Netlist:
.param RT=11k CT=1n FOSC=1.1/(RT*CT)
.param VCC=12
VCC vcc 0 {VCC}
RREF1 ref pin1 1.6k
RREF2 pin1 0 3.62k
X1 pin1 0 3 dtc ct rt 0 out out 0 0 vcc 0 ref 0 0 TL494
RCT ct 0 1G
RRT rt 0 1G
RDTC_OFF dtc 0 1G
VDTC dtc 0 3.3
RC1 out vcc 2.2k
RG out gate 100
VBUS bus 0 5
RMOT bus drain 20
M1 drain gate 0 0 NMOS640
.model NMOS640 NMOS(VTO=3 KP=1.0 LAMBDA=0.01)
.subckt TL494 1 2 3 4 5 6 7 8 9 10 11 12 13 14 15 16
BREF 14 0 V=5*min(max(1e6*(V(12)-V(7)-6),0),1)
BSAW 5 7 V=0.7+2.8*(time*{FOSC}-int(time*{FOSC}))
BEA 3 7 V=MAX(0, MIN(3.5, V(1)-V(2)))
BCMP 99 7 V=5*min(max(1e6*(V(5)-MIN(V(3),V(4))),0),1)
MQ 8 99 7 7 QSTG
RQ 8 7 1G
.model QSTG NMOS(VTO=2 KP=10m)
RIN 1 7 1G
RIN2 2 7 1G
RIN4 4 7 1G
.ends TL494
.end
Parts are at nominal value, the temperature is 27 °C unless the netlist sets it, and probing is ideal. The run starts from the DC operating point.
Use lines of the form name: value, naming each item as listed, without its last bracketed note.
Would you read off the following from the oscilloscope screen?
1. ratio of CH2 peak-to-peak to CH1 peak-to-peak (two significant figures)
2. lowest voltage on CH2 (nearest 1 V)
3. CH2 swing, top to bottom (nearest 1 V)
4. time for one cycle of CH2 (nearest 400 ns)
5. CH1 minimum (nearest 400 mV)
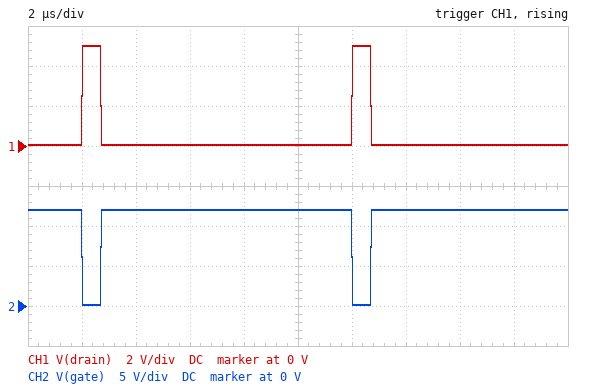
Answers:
ratio of CH2 peak-to-peak to CH1 peak-to-peak: 2.4
lowest voltage on CH2: 0 V
CH2 swing, top to bottom: 12 V
time for one cycle of CH2: 10.0 µs
CH1 minimum: 0 V
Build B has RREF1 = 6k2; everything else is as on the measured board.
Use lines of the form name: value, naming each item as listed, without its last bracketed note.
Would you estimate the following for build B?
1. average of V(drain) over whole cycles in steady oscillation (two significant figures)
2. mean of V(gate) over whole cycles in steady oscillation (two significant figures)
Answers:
average of V(drain) over whole cycles in steady oscillation: 3.0 V
mean of V(gate) over whole cycles in steady oscillation: 5.0 V
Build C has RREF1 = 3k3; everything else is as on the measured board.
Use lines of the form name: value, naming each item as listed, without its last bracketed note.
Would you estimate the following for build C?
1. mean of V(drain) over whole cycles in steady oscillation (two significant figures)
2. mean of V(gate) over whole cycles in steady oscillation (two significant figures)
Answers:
mean of V(drain) over whole cycles in steady oscillation: 1.6 V
mean of V(gate) over whole cycles in steady oscillation: 8.3 V
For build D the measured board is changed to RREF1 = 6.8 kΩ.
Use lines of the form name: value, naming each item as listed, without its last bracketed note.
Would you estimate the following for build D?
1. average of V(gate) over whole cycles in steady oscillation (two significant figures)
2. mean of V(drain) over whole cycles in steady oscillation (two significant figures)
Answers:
average of V(gate) over whole cycles in steady oscillation: 4.6 V
mean of V(drain) over whole cycles in steady oscillation: 3.2 V
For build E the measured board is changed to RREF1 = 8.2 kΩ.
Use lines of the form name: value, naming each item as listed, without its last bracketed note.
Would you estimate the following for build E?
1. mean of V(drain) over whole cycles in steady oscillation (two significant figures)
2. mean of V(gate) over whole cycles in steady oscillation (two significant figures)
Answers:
mean of V(drain) over whole cycles in steady oscillation: 3.5 V
mean of V(gate) over whole cycles in steady oscillation: 3.7 V
